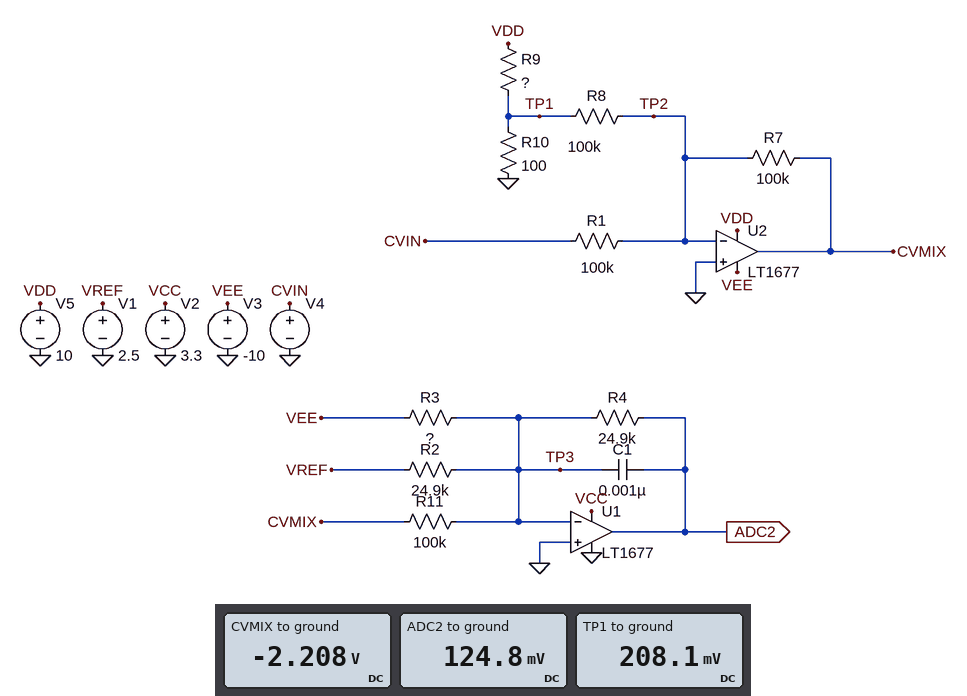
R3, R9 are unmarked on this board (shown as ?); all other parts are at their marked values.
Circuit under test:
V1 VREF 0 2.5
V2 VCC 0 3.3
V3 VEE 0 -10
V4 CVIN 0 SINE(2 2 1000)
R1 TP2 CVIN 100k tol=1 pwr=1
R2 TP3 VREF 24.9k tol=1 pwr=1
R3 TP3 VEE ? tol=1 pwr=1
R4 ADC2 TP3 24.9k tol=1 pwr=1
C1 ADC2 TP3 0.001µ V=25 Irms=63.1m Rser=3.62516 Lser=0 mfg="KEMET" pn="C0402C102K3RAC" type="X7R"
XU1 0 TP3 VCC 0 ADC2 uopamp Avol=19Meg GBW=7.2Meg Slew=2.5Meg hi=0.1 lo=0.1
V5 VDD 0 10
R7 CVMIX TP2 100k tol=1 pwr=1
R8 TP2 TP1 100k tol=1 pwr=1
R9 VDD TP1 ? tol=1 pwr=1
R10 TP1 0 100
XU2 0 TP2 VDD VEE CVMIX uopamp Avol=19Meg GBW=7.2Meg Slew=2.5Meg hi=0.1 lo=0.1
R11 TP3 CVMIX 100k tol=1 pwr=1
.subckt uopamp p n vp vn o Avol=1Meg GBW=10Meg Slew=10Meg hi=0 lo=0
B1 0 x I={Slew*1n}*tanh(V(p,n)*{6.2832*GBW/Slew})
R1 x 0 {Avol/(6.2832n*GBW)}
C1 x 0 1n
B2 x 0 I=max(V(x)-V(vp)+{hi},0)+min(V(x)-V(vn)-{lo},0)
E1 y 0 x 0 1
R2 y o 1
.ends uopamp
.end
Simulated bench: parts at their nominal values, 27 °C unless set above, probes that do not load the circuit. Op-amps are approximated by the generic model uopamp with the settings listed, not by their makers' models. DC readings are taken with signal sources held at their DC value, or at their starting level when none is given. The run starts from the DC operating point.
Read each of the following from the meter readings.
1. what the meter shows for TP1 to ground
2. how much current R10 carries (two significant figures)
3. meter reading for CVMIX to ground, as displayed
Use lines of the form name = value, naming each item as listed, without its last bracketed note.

what the meter shows for TP1 to ground = 208.1 mV
how much current R10 carries = 2.1 mA
meter reading for CVMIX to ground, as displayed = -2.208 V
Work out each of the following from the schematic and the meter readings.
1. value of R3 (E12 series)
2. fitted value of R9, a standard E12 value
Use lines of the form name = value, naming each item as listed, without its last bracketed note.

value of R3 = 120 kΩ
fitted value of R9, a standard E12 value = 4.7 kΩ
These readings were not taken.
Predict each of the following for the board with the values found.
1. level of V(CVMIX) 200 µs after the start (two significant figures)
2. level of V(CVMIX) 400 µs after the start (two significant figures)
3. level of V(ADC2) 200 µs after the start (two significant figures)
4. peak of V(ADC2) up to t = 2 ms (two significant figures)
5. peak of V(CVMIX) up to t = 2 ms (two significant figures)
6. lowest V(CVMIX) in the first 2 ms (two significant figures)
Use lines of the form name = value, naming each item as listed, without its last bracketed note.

level of V(CVMIX) 200 µs after the start = -4.1 V
level of V(CVMIX) 400 µs after the start = -3.4 V
level of V(ADC2) 200 µs after the start = 560 mV
peak of V(ADC2) up to t = 2 ms = 620 mV
peak of V(CVMIX) up to t = 2 ms = -210 mV
lowest V(CVMIX) in the first 2 ms = -4.2 V
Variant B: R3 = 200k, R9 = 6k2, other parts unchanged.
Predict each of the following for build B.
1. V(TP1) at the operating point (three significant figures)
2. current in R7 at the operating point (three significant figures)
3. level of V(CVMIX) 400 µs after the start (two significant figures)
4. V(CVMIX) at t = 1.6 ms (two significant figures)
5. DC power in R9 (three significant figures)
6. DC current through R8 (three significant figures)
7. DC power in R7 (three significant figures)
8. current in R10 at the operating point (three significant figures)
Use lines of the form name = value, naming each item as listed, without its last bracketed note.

V(TP1) at the operating point = 159 mV
current in R7 at the operating point = 21.6 µA
level of V(CVMIX) 400 µs after the start = -3.3 V
V(CVMIX) at t = 1.6 ms = -980 mV
DC power in R9 = 15.6 mW
DC current through R8 = 1.59 µA
DC power in R7 = 46.6 µW
current in R10 at the operating point = 1.59 mA
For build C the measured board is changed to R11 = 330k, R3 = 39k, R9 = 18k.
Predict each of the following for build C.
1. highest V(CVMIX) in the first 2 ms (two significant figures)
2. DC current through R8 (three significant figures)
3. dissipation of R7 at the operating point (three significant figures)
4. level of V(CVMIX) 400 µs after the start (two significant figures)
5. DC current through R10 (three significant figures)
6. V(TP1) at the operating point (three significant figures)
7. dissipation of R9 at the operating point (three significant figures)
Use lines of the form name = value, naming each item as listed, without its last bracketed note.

highest V(CVMIX) in the first 2 ms = -55 mV
DC current through R8 = 552 nA
dissipation of R7 at the operating point = 42.2 µW
level of V(CVMIX) 400 µs after the start = -3.2 V
DC current through R10 = 552 µA
V(TP1) at the operating point = 55.2 mV
dissipation of R9 at the operating point = 5.49 mW
